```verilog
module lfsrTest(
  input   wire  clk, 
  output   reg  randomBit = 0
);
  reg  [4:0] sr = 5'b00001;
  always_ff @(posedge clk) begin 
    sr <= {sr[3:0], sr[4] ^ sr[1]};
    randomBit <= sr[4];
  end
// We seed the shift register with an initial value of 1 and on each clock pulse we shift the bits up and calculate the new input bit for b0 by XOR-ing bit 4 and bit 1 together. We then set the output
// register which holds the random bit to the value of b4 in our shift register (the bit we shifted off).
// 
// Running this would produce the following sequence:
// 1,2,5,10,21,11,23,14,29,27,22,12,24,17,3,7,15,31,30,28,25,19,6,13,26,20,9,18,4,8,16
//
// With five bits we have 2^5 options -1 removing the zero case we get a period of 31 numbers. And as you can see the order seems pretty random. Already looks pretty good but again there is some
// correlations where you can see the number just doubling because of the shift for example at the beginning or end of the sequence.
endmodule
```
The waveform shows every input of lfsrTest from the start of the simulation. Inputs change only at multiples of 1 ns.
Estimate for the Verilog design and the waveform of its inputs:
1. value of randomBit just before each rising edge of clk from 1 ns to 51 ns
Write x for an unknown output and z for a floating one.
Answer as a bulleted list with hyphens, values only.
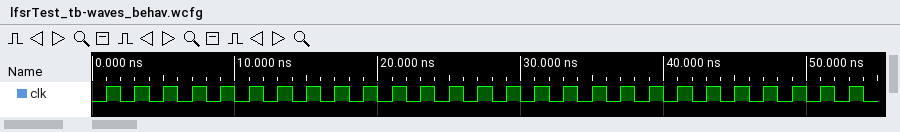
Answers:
- 0 0 0 0 0 1 0 1 0 1 1 1 0 1 1 0 0 0 1 1 1 1 1 0 0 1
